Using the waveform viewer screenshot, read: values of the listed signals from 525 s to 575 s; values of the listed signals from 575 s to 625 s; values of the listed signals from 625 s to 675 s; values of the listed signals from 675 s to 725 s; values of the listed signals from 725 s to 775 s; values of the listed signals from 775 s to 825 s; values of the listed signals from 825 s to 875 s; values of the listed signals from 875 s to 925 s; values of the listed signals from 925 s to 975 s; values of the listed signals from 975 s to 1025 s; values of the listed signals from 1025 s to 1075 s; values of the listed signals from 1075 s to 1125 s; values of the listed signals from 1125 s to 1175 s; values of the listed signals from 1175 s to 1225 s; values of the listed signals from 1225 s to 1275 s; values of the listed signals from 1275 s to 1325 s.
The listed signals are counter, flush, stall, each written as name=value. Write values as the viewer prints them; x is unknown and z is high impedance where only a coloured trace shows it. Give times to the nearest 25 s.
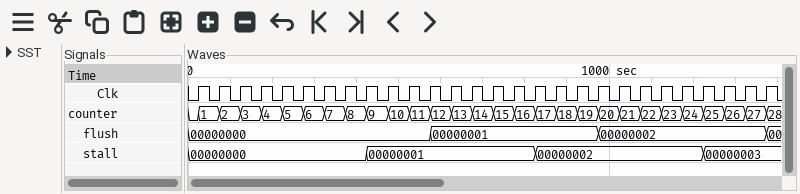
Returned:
counter=11, flush=00000000, stall=00000001
counter=12, flush=00000001, stall=00000001
counter=13, flush=00000001, stall=00000001
counter=14, flush=00000001, stall=00000001
counter=15, flush=00000001, stall=00000001
counter=16, flush=00000001, stall=00000001
counter=17, flush=00000001, stall=00000002
counter=18, flush=00000001, stall=00000002
counter=19, flush=00000001, stall=00000002
counter=20, flush=00000002, stall=00000002
counter=21, flush=00000002, stall=00000002
counter=22, flush=00000002, stall=00000002
counter=23, flush=00000002, stall=00000002
counter=24, flush=00000002, stall=00000002
counter=25, flush=00000002, stall=00000003
counter=26, flush=00000002, stall=00000003
